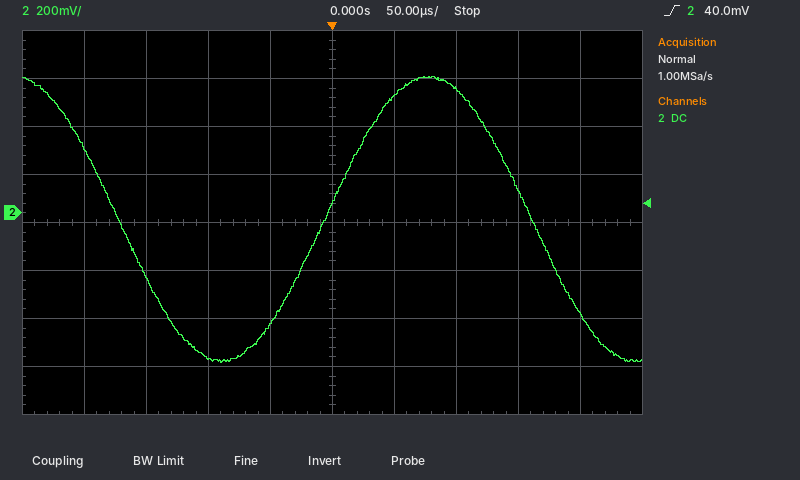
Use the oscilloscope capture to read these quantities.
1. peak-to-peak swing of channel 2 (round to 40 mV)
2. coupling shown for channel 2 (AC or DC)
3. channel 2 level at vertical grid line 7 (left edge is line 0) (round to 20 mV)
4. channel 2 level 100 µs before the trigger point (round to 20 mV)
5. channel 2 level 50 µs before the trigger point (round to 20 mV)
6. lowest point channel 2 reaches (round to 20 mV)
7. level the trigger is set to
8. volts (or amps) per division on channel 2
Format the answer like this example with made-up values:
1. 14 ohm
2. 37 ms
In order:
1. 1.20 V
2. DC
3. 520 mV
4. -600 mV
5. -460 mV
6. -620 mV
7. 40.0 mV
8. 200 mV
